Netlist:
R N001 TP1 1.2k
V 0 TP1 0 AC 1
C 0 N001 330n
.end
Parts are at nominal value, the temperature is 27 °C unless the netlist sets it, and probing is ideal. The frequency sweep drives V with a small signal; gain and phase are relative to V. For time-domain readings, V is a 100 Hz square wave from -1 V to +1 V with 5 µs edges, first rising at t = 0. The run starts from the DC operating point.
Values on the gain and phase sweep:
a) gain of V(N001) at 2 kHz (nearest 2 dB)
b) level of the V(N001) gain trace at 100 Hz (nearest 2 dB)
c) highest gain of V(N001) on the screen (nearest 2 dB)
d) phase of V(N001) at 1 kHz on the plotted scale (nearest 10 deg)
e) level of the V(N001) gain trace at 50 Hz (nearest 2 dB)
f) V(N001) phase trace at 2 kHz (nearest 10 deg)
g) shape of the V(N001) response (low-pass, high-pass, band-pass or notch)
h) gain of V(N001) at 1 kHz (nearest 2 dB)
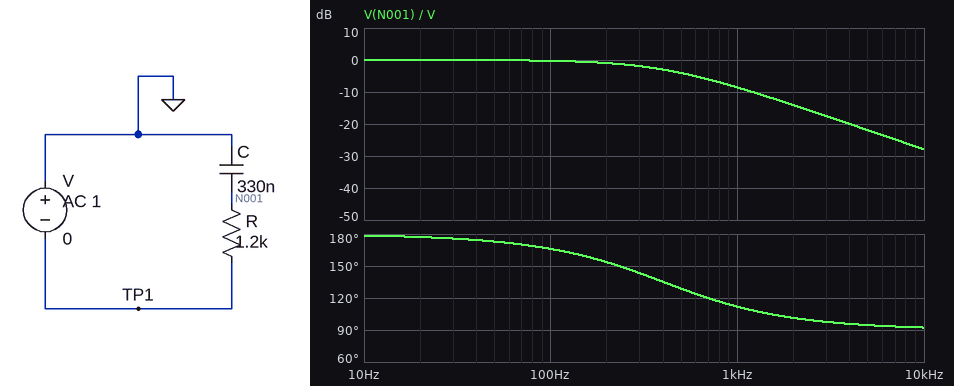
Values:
-14 dB
0 dB
0 dB
110 deg
0 dB
100 deg
low-pass
-8 dB
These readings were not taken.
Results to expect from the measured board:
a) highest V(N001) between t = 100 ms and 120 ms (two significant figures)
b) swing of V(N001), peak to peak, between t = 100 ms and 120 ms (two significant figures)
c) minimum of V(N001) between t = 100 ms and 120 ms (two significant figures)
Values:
1.0 V
2.0 V
-1.0 V
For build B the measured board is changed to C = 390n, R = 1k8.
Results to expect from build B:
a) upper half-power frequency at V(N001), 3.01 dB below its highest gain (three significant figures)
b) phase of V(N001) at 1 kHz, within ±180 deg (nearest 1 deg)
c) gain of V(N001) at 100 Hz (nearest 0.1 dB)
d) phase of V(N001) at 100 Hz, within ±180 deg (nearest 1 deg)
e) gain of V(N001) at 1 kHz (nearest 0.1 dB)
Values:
227 Hz
103 deg
-0.8 dB
156 deg
-13.1 dB
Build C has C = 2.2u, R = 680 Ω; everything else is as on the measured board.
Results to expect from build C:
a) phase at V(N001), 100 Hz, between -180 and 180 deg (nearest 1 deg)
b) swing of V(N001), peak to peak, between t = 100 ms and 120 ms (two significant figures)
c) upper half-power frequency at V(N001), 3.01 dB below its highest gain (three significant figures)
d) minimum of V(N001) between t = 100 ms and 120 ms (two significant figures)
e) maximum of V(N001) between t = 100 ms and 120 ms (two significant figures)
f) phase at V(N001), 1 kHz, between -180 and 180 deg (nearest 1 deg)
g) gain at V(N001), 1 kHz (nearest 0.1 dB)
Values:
137 deg
1.9 V
106 Hz
-930 mV
930 mV
96 deg
-19.5 dB
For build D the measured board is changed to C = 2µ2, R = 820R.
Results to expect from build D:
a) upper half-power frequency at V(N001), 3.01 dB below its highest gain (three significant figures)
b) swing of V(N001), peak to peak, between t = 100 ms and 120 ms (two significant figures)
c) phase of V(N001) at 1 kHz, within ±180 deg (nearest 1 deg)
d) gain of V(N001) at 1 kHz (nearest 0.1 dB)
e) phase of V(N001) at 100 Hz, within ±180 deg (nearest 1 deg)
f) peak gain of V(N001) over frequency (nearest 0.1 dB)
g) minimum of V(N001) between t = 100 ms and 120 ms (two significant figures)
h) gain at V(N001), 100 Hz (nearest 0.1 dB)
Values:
88.2 Hz
1.8 V
95 deg
-21.1 dB
131 deg
0 dB
-880 mV
-3.6 dB
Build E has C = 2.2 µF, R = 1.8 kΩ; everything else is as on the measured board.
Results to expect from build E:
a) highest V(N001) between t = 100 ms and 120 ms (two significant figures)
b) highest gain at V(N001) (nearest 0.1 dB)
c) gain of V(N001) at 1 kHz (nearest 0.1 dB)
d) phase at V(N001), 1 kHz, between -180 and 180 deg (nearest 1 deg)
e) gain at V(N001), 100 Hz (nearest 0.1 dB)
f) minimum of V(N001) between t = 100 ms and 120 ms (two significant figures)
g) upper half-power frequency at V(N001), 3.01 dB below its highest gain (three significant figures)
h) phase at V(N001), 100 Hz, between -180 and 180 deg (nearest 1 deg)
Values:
560 mV
0 dB
-27.9 dB
92 deg
-8.6 dB
-560 mV
40.2 Hz
112 deg
